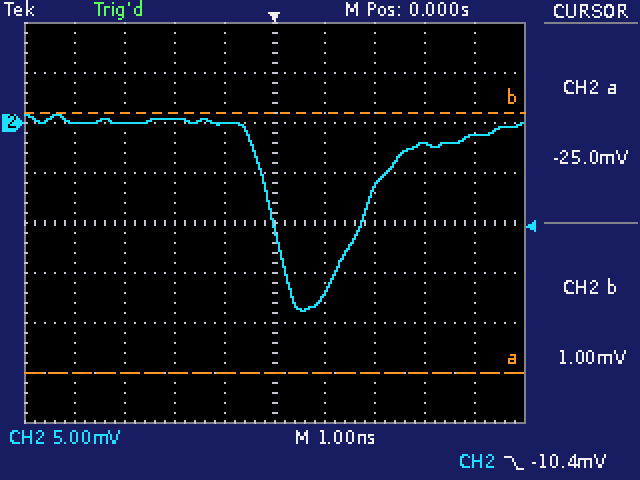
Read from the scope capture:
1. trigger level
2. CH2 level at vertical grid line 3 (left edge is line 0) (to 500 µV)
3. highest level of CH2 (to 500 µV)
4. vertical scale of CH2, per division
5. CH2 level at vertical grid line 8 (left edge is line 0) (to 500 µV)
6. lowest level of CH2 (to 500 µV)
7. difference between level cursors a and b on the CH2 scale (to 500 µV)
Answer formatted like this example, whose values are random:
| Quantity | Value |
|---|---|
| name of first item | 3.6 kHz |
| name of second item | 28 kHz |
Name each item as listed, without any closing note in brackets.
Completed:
| Quantity | Value |
|---|---|
| trigger level | -10.4 mV |
| CH2 level at vertical grid line 3 (left edge is line 0) | 500 µV |
| highest level of CH2 | 1.0 mV |
| vertical scale of CH2, per division | 5 mV |
| CH2 level at vertical grid line 8 (left edge is line 0) | -2.0 mV |
| lowest level of CH2 | -19.0 mV |
| difference between level cursors a and b on the CH2 scale | 26.0 mV |
